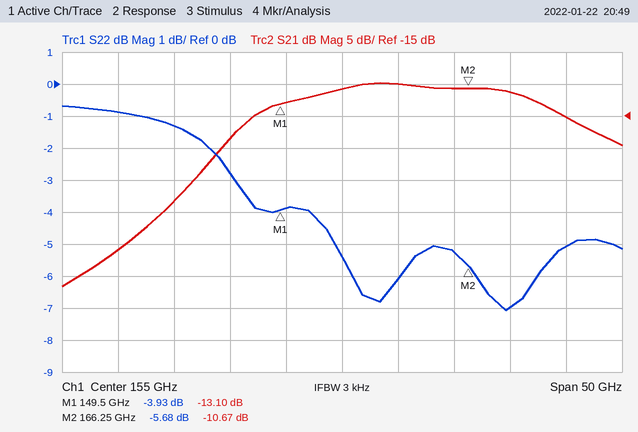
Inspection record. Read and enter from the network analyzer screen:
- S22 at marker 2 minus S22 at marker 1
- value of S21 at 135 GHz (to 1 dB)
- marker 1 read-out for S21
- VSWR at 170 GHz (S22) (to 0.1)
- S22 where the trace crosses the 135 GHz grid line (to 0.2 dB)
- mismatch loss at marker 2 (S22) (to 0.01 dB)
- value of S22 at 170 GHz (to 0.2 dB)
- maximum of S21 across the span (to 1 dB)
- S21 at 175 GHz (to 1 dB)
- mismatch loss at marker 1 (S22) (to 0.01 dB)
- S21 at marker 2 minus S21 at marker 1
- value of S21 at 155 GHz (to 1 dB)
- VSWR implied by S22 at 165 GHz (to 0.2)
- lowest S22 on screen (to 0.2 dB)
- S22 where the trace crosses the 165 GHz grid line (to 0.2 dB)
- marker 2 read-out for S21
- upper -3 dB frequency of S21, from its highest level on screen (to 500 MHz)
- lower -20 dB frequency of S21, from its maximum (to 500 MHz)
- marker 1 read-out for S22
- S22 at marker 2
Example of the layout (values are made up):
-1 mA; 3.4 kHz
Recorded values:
-1.75 dB; -36 dB; -13.10 dB; 2.6; -0.8 dB; 1.37 dB; -7.0 dB; -10 dB; -15 dB; 2.25 dB; 2.43 dB; -11 dB; 3.4; -7.0 dB; -5.2 dB; -10.67 dB; 172.5 GHz; 139.0 GHz; -3.93 dB; -5.68 dB
